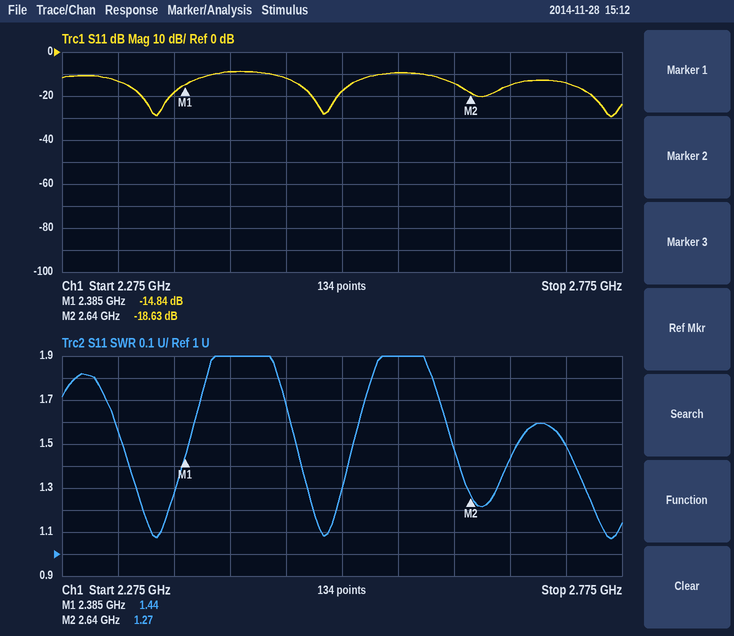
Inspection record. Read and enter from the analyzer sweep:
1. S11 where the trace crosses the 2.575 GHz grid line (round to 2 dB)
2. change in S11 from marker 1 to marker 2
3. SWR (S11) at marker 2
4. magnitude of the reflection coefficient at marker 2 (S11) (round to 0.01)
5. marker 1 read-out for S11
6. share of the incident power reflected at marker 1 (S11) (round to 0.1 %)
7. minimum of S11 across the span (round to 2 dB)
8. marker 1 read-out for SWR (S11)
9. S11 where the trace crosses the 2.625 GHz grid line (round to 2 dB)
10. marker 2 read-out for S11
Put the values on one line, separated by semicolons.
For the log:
-10 dB; -3.79 dB; 1.27; 0.12; -14.84 dB; 3.3 %; -30 dB; 1.44; -14 dB; -18.63 dB
